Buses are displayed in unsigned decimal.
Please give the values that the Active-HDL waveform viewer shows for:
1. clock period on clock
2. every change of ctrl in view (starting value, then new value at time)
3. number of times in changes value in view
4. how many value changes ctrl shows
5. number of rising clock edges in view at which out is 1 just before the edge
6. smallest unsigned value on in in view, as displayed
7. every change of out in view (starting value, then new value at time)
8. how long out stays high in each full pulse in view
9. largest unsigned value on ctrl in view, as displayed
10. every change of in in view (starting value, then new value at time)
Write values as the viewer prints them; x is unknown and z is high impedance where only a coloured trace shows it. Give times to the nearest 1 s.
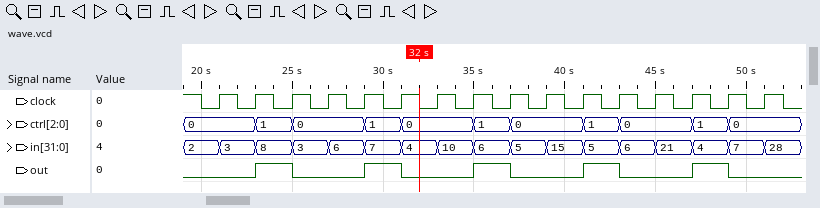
2 s
0, 1 at 23 s, 0 at 25 s, 1 at 29 s, 0 at 31 s, 1 at 35 s, 0 at 37 s, 1 at 41 s, 0 at 43 s, 1 at 47 s, 0 at 49 s
16
10
5
2
0, 1 at 23 s, 0 at 25 s, 1 at 29 s, 0 at 31 s, 1 at 35 s, 0 at 37 s, 1 at 41 s, 0 at 43 s, 1 at 47 s, 0 at 49 s
2 s, 2 s, 2 s, 2 s, 2 s
1
2, 3 at 21 s, 8 at 23 s, 3 at 25 s, 6 at 27 s, 7 at 29 s, 4 at 31 s, 10 at 33 s, 6 at 35 s, 5 at 37 s, 15 at 39 s, 5 at 41 s, 6 at 43 s, 21 at 45 s, 4 at 47 s, 7 at 49 s, 28 at 51 s
